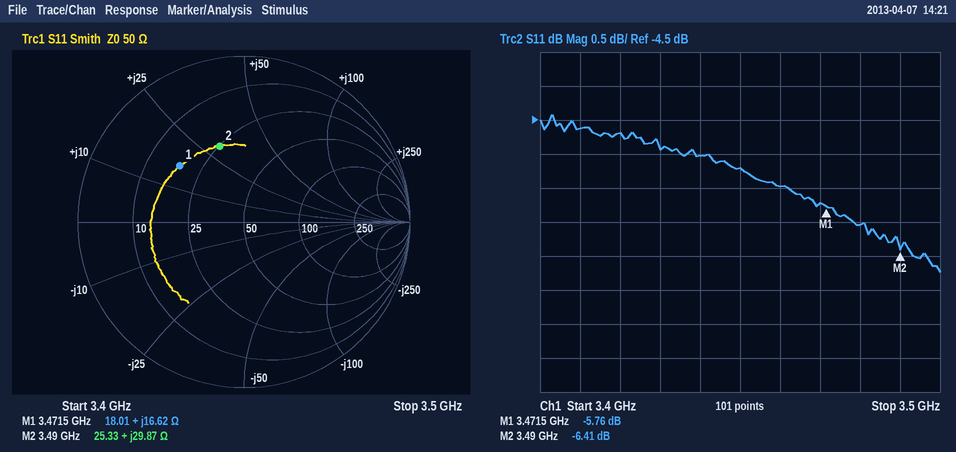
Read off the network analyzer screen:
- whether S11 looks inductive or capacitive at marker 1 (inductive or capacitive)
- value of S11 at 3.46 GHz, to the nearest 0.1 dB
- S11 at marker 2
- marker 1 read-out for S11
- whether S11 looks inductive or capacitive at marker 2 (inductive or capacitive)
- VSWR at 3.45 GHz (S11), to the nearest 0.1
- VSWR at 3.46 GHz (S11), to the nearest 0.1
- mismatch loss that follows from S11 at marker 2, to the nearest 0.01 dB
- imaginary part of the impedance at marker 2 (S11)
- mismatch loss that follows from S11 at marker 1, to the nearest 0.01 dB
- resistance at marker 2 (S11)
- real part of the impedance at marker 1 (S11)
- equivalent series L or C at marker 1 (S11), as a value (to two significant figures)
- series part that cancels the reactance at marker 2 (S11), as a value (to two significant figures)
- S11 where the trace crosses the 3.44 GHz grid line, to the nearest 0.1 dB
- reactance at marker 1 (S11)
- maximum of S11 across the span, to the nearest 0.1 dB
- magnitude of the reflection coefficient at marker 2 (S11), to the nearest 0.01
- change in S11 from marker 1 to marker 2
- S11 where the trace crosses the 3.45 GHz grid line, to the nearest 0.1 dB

inductive
-5.5 dB
-6.41 dB
-5.76 dB
inductive
3.4
3.3
1.13 dB
+29.87 Ω
1.34 dB
25.33 Ω
18.01 Ω
760 pH
1.5 pF
-5.0 dB
+16.62 Ω
-4.4 dB
0.48
-0.65 dB
-5.2 dB
